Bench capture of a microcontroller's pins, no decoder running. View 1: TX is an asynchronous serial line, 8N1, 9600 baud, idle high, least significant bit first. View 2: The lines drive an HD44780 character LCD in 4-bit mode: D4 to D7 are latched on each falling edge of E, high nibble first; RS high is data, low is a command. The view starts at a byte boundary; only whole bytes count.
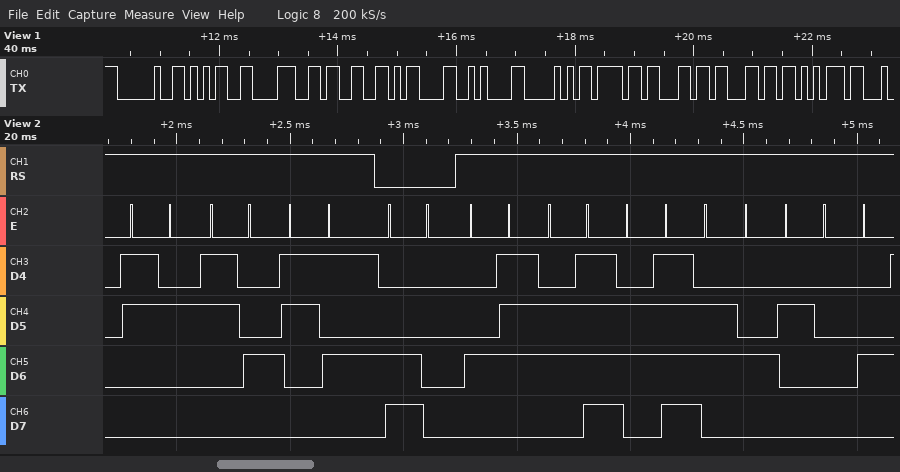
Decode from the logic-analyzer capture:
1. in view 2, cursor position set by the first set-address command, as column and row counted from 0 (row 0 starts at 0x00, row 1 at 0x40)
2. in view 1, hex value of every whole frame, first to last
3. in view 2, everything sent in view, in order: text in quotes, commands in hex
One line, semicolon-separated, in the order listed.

column 0, row 1; 20 35 38 33 0D 0A 50 6F 6C 6C 75; "245" 0xC0 "Good "
